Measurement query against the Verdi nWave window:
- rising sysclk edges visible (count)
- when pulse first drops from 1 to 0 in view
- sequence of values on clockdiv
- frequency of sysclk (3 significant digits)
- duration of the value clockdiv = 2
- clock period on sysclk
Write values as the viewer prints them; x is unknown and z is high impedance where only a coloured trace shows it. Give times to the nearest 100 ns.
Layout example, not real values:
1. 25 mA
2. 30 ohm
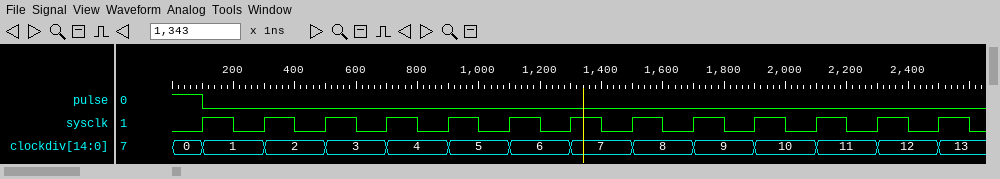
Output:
1. 13
2. 100 ns
3. 0, 1, 2, 3, 4, 5, 6, 7, 8, 9, 10, 11, 12, 13
4. 5.00 MHz
5. 200 ns
6. 200 ns
